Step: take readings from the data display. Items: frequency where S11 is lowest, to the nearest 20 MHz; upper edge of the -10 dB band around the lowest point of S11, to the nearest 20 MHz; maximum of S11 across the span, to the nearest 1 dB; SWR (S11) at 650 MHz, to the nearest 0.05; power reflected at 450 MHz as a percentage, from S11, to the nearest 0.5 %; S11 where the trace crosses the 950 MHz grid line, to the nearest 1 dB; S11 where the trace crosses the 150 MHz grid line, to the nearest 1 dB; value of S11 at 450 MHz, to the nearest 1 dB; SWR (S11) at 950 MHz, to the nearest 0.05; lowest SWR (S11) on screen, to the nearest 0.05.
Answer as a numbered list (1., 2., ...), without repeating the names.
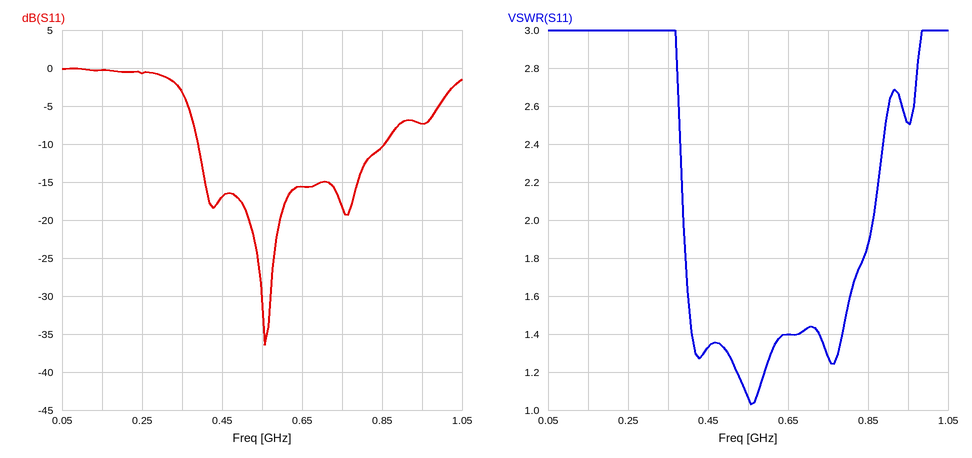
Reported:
1. 560 MHz
2. 860 MHz
3. 0 dB
4. 1.40
5. 2.0 %
6. -7 dB
7. 0 dB
8. -17 dB
9. 2.50
10. 1.05
